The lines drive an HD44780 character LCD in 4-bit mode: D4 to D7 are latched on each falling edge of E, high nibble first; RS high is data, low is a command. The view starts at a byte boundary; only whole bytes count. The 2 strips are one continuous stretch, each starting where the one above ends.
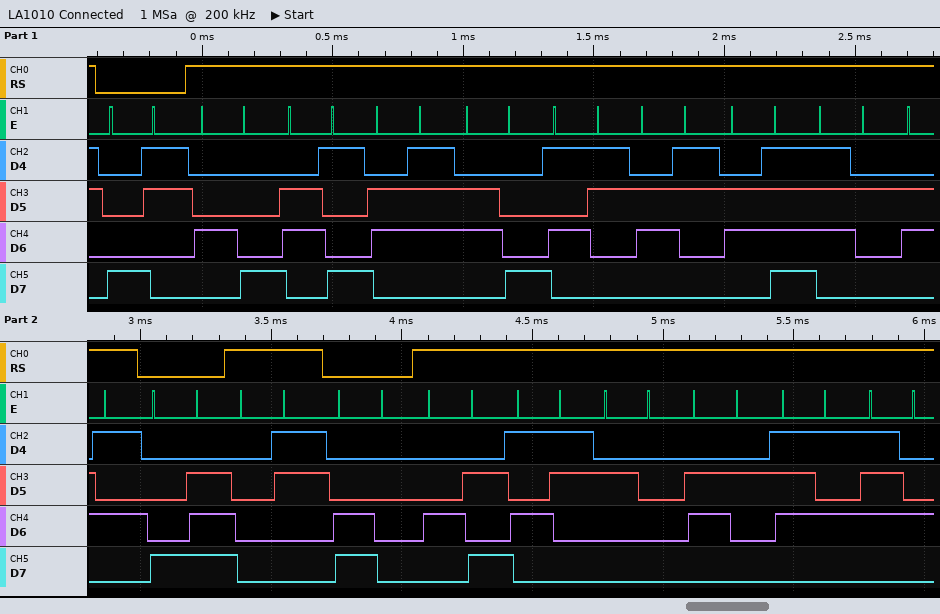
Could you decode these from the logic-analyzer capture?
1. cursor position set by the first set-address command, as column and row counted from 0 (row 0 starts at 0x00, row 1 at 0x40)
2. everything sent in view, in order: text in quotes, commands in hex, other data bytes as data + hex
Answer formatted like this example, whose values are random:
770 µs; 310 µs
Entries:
column 3, row 0; 0x83 "HighScore" 0x8E data 03 0xC0 "JS but"
